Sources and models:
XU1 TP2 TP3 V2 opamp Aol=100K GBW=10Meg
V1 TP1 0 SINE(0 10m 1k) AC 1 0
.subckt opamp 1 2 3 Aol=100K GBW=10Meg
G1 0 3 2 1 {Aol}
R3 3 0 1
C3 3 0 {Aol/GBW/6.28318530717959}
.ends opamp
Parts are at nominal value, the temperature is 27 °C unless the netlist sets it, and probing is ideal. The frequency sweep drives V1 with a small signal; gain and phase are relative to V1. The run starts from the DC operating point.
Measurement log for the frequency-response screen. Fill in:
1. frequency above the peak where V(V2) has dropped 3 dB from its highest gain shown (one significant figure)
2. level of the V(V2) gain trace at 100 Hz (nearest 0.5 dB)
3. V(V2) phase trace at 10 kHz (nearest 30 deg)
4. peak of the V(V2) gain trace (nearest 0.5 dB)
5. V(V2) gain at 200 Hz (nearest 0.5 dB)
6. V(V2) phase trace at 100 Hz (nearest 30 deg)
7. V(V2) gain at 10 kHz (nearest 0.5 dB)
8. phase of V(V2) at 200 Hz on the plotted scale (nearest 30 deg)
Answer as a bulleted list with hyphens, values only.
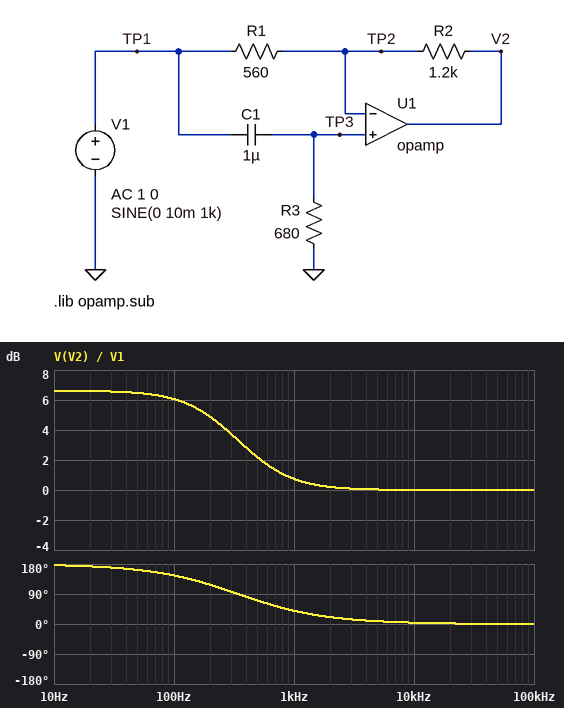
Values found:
- 300 Hz
- 6.0 dB
- 0 deg
- 6.5 dB
- 5.0 dB
- 150 deg
- 0 dB
- 120 deg
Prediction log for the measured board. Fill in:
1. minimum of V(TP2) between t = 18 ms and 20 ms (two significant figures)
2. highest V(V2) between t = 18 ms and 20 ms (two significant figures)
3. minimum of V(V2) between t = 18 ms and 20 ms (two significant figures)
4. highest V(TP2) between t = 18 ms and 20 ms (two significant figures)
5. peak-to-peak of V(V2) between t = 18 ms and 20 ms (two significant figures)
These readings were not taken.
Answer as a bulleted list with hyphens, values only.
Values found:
- -9.7 mV
- 11 mV
- -11 mV
- 9.7 mV
- 22 mV
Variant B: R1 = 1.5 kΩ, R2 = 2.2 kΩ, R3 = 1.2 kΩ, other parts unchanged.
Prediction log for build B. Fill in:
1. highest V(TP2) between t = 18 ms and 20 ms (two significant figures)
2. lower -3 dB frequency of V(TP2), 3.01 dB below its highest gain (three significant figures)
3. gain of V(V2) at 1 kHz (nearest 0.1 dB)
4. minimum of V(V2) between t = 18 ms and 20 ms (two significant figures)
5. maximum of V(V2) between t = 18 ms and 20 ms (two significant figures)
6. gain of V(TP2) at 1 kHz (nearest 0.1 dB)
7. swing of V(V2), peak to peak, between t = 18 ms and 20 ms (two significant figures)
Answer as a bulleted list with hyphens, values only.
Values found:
- 9.9 mV
- 133 Hz
- 0.1 dB
- -10 mV
- 10 mV
- -0.1 dB
- 20 mV
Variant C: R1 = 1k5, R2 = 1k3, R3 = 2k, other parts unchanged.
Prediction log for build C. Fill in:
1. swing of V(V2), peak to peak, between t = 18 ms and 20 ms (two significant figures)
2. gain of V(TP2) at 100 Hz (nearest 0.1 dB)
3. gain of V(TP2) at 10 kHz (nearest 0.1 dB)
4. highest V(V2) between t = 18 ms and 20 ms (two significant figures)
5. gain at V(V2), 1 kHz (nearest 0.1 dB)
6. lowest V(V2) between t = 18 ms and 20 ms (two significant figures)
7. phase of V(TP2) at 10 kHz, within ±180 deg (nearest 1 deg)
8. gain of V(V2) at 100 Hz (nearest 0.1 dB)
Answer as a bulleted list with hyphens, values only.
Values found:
- 20 mV
- -2.1 dB
- 0 dB
- 10 mV
- 0 dB
- -10 mV
- 0 deg
- -0.4 dB
